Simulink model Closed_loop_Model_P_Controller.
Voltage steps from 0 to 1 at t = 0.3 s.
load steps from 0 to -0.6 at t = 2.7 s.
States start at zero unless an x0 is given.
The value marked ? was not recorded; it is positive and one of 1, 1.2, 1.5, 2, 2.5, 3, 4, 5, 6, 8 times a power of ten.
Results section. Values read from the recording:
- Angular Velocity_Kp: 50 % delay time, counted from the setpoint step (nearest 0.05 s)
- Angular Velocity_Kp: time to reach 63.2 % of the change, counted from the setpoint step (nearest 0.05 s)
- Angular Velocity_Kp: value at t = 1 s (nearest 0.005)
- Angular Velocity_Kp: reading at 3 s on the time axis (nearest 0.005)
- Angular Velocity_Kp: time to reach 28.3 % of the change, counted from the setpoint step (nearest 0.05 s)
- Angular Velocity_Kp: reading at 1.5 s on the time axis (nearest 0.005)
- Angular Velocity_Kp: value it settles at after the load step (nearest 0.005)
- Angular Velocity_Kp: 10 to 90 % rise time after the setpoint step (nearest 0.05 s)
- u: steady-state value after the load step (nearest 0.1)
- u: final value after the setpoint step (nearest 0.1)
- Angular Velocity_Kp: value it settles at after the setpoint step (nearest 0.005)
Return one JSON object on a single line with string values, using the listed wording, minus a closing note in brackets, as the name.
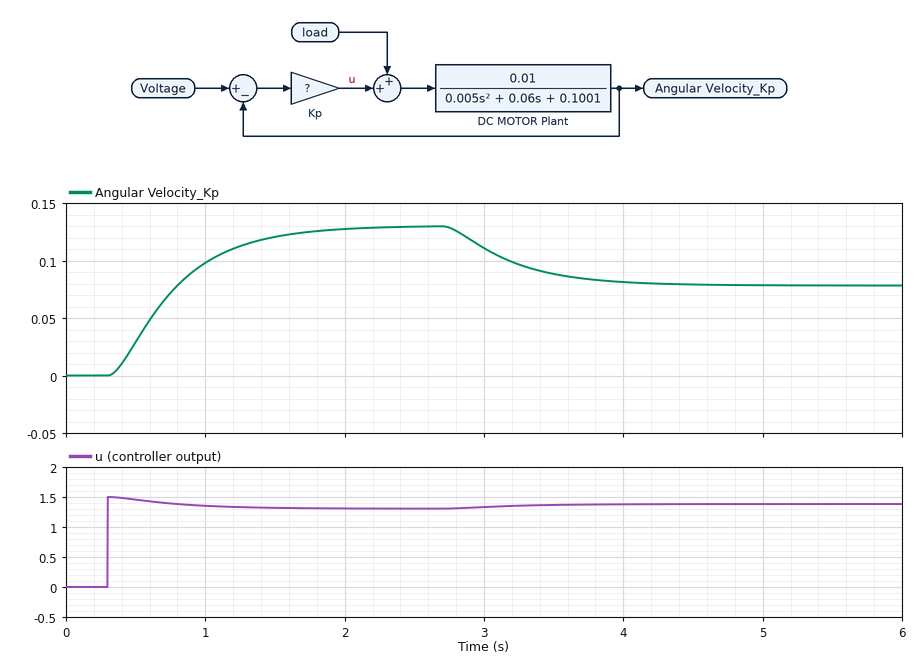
{"Angular Velocity_Kp: 50 % delay time, counted from the setpoint step": "0.40 s", "Angular Velocity_Kp: time to reach 63.2 % of the change, counted from the setpoint step": "0.55 s", "Angular Velocity_Kp: value at t = 1 s": "0.100", "Angular Velocity_Kp: reading at 3 s on the time axis": "0.110", "Angular Velocity_Kp: time to reach 28.3 % of the change, counted from the setpoint step": "0.25 s", "Angular Velocity_Kp: reading at 1.5 s on the time axis": "0.120", "Angular Velocity_Kp: value it settles at after the load step": "0.080", "Angular Velocity_Kp: 10 to 90 % rise time after the setpoint step": "0.95 s", "u: steady-state value after the load step": "1.4", "u: final value after the setpoint step": "1.3", "Angular Velocity_Kp: value it settles at after the setpoint step": "0.130"}
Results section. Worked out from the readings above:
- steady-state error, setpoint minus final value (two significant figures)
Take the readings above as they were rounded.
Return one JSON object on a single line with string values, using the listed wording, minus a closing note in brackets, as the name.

{"steady-state error, setpoint minus final value": "0.87"}
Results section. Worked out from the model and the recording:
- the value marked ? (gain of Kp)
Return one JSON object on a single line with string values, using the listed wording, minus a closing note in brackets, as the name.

{"the value marked ?": "1.5"}
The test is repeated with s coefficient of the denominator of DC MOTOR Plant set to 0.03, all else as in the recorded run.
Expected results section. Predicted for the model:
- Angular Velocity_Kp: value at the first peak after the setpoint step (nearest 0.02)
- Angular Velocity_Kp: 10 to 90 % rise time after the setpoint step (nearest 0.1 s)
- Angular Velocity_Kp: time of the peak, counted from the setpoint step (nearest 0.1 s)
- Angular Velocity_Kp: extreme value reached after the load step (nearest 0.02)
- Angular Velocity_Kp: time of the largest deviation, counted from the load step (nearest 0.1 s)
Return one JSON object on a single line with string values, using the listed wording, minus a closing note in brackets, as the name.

{"Angular Velocity_Kp: value at the first peak after the setpoint step": "0.14", "Angular Velocity_Kp: 10 to 90 % rise time after the setpoint step": "0.4 s", "Angular Velocity_Kp: time of the peak, counted from the setpoint step": "0.8 s", "Angular Velocity_Kp: extreme value reached after the load step": "0.08", "Angular Velocity_Kp: time of the largest deviation, counted from the load step": "0.8 s"}
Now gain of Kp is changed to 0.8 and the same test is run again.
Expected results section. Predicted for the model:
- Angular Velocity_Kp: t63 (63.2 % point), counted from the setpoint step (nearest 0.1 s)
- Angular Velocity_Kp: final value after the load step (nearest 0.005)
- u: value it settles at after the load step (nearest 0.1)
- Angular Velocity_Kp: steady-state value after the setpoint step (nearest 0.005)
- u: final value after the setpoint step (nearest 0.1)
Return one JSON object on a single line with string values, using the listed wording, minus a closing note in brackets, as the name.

{"Angular Velocity_Kp: t63 (63.2 % point), counted from the setpoint step": "0.6 s", "Angular Velocity_Kp: final value after the load step": "0.020", "u: value it settles at after the load step": "0.8", "Angular Velocity_Kp: steady-state value after the setpoint step": "0.075", "u: final value after the setpoint step": "0.7"}
